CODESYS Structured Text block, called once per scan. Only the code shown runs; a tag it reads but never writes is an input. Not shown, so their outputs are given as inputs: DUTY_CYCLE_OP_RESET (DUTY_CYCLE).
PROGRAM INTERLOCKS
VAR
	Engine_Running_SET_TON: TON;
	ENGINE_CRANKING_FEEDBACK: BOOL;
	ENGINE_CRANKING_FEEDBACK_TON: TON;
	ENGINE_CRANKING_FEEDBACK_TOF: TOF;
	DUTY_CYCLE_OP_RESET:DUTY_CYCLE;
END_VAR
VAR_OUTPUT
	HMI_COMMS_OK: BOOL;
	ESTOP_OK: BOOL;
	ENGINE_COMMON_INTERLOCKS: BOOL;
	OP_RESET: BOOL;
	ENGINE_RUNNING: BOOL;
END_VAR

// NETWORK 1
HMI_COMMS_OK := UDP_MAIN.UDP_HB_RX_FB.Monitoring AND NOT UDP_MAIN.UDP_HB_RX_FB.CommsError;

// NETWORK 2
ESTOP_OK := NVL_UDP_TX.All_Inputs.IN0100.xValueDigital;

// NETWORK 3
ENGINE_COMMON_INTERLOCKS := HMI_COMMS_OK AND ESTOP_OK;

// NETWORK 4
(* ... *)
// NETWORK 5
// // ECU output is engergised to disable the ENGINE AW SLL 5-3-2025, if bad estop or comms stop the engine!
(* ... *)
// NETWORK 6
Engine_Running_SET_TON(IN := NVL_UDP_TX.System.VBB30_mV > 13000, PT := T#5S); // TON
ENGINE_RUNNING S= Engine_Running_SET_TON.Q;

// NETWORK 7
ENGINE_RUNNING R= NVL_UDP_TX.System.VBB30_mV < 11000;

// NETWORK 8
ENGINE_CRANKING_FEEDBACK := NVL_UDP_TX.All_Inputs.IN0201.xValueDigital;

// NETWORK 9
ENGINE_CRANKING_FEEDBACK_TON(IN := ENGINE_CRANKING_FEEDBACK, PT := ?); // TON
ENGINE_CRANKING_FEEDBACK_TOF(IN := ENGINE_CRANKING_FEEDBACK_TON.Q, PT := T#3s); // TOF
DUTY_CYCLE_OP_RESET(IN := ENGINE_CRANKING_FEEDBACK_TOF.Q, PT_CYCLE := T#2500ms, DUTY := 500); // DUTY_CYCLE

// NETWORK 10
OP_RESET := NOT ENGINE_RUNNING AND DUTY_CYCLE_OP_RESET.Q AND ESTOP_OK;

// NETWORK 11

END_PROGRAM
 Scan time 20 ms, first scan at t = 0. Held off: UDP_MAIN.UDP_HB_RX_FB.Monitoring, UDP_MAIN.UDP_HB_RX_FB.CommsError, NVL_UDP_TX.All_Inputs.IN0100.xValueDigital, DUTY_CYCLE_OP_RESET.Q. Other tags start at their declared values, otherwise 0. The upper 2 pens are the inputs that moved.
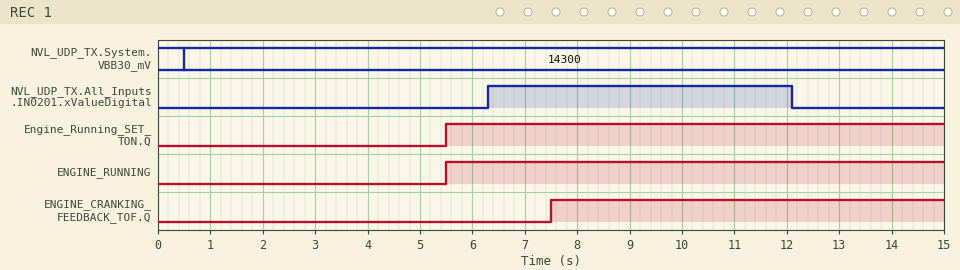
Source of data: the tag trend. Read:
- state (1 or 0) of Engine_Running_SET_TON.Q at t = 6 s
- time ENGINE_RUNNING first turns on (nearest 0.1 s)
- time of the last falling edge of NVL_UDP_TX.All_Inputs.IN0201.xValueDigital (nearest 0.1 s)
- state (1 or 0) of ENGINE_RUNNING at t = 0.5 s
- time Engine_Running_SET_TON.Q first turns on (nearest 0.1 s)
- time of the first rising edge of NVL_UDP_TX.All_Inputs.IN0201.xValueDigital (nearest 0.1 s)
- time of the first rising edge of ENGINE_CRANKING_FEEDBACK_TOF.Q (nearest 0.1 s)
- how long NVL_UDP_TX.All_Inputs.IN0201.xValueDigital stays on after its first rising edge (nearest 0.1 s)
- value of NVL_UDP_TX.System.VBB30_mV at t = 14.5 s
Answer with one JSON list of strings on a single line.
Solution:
["1", "5.5 s", "12.1 s", "0", "5.5 s", "6.3 s", "7.5 s", "5.8 s", "14300"]
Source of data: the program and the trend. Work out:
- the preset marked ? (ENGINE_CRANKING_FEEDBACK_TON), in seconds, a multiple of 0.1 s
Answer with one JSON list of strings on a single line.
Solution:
["1.2 s"]
